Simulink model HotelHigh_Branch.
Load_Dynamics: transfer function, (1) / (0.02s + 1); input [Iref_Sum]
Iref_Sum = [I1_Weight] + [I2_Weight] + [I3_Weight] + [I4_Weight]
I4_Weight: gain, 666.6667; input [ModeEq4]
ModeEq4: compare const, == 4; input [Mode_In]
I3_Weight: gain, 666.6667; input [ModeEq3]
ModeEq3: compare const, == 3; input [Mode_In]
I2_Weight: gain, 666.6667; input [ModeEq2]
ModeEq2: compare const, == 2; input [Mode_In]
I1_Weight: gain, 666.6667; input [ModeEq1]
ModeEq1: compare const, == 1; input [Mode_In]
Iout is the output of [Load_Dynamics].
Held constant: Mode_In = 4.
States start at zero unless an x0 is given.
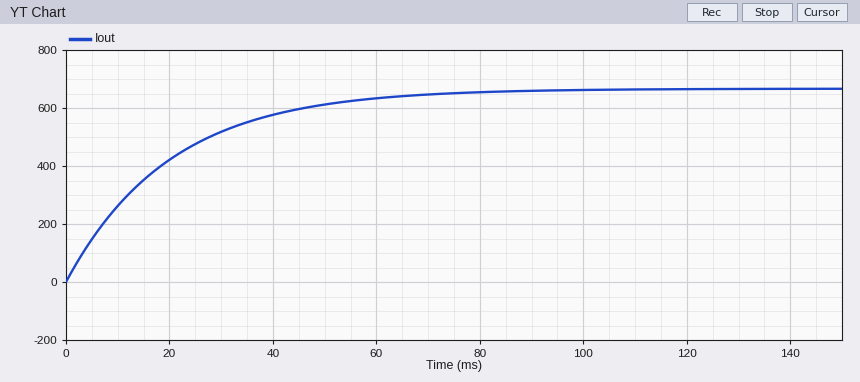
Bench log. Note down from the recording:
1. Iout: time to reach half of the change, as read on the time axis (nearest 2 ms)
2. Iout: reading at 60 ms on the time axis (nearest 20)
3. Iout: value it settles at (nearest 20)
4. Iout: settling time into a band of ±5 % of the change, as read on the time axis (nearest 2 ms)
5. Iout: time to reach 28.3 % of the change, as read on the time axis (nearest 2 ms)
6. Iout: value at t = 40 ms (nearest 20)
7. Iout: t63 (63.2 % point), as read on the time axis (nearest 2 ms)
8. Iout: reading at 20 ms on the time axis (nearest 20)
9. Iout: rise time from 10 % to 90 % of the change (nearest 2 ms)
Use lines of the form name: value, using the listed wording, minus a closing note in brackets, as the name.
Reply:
Iout: time to reach half of the change, as read on the time axis: 14 ms
Iout: reading at 60 ms on the time axis: 640
Iout: value it settles at: 660
Iout: settling time into a band of ±5 % of the change, as read on the time axis: 60 ms
Iout: time to reach 28.3 % of the change, as read on the time axis: 6 ms
Iout: value at t = 40 ms: 580
Iout: t63 (63.2 % point), as read on the time axis: 20 ms
Iout: reading at 20 ms on the time axis: 420
Iout: rise time from 10 % to 90 % of the change: 44 ms
